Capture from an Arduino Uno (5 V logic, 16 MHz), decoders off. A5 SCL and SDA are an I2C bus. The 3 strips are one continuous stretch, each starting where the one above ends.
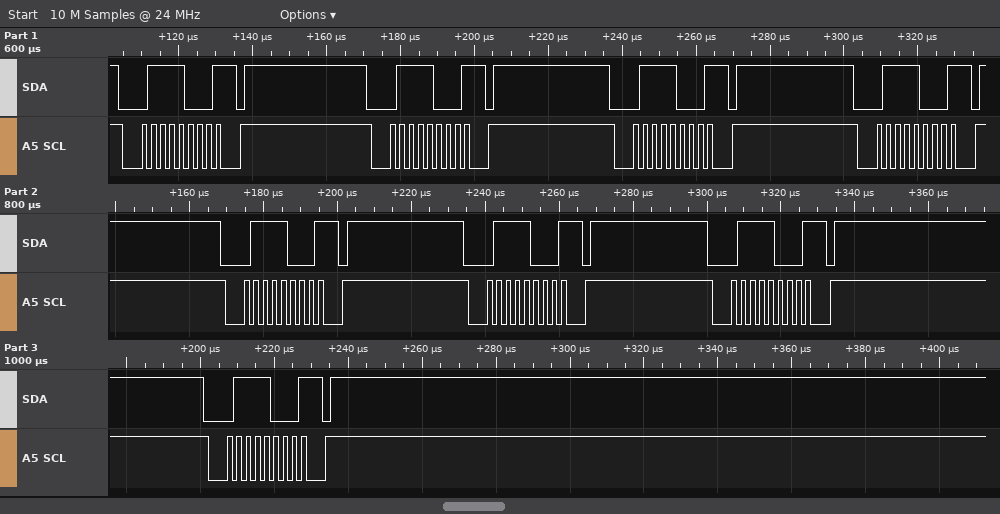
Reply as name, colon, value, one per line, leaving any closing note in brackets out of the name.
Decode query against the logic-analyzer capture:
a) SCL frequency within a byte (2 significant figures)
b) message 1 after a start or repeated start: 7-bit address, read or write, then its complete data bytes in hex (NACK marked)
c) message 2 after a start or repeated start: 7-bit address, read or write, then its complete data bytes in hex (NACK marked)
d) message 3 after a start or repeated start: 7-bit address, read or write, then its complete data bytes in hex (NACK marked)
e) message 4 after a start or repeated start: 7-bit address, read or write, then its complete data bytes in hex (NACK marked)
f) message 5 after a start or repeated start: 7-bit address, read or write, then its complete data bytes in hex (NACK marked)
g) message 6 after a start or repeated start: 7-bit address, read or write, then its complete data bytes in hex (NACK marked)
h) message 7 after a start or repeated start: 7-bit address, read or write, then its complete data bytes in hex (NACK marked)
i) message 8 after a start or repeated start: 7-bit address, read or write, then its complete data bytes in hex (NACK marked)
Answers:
SCL frequency within a byte: 400 kHz
message 1 after a start or repeated start: 7-bit address, read or write, then its complete data bytes in hex: 0x3C write NACK
message 2 after a start or repeated start: 7-bit address, read or write, then its complete data bytes in hex: 0x3C write NACK
message 3 after a start or repeated start: 7-bit address, read or write, then its complete data bytes in hex: 0x3C write NACK
message 4 after a start or repeated start: 7-bit address, read or write, then its complete data bytes in hex: 0x3C write NACK
message 5 after a start or repeated start: 7-bit address, read or write, then its complete data bytes in hex: 0x3C write NACK
message 6 after a start or repeated start: 7-bit address, read or write, then its complete data bytes in hex: 0x3C write NACK
message 7 after a start or repeated start: 7-bit address, read or write, then its complete data bytes in hex: 0x3C write NACK
message 8 after a start or repeated start: 7-bit address, read or write, then its complete data bytes in hex: 0x3C write NACK
